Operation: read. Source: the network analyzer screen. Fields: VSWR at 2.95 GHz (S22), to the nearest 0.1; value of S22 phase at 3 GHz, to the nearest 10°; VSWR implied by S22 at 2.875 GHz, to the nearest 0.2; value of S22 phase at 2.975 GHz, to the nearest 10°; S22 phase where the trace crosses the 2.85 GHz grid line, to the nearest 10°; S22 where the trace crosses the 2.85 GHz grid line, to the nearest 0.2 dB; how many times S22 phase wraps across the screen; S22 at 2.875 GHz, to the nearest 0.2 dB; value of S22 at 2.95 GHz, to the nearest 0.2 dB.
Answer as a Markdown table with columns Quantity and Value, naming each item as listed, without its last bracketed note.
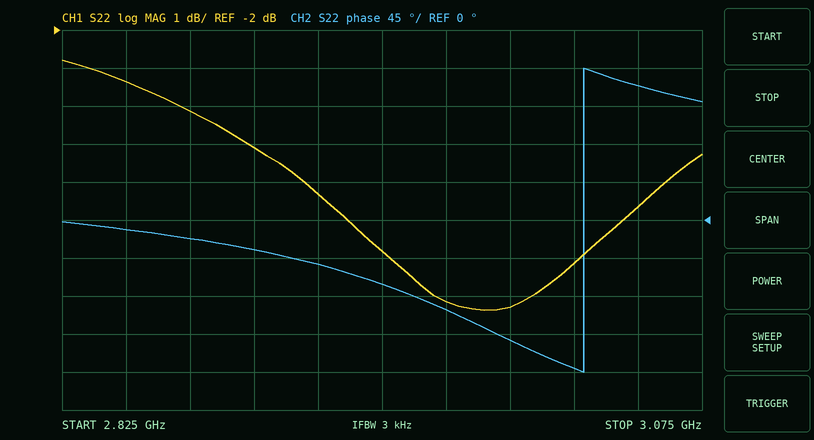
| Quantity | Value |
|---|---|
| VSWR at 2.95 GHz (S22), to the nearest 0.1 | 2.4 |
| value of S22 phase at 3 GHz, to the nearest 10° | -140° |
| VSWR implied by S22 at 2.875 GHz, to the nearest 0.2 | 4.2 |
| value of S22 phase at 2.975 GHz, to the nearest 10° | -110° |
| S22 phase where the trace crosses the 2.85 GHz grid line, to the nearest 10° | -10° |
| S22 where the trace crosses the 2.85 GHz grid line, to the nearest 0.2 dB | -3.4 dB |
| how many times S22 phase wraps across the screen | 1 |
| S22 at 2.875 GHz, to the nearest 0.2 dB | -4.2 dB |
| value of S22 at 2.95 GHz, to the nearest 0.2 dB | -7.8 dB |
